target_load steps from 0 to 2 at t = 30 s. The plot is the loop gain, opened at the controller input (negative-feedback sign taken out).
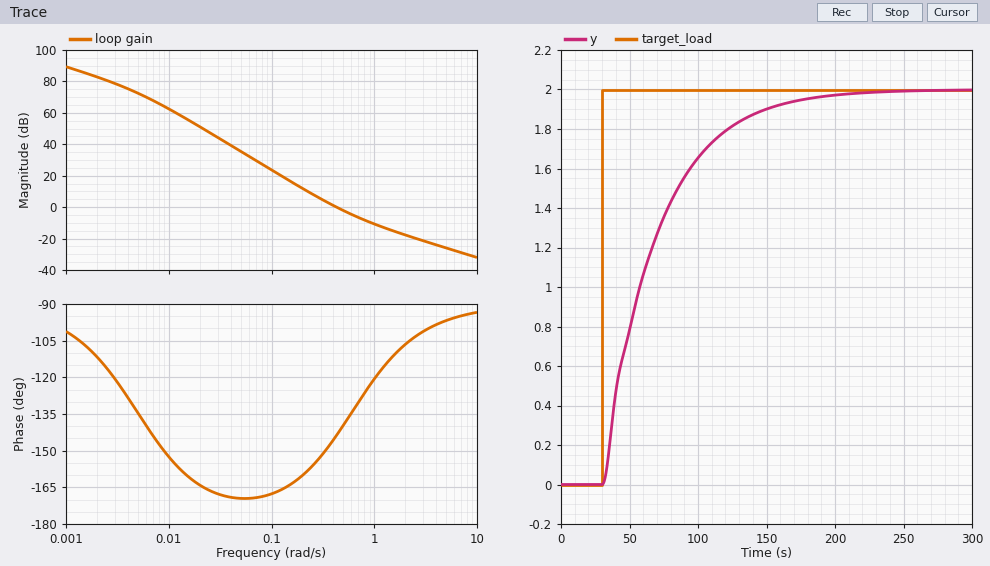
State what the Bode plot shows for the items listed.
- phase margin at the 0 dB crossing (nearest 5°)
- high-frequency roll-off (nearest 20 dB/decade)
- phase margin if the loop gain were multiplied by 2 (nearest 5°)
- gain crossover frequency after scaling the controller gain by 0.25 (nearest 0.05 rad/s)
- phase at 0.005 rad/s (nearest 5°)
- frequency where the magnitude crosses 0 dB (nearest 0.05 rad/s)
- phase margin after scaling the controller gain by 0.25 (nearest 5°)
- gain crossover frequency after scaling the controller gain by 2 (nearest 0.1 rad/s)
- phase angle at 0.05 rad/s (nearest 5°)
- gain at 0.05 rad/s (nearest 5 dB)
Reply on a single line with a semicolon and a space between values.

35°; -20 dB/decade; 50°; 0.20 rad/s; -135°; 0.45 rad/s; 20°; 0.7 rad/s; -170°; 35 dB
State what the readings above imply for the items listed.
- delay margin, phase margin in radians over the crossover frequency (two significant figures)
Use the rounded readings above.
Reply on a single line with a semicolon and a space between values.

1.4 s
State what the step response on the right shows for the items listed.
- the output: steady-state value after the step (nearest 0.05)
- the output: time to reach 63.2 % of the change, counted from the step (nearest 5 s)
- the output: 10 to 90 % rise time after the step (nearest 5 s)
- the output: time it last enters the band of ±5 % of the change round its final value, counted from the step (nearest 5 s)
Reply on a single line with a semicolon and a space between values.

2.00; 40 s; 85 s; 120 s
